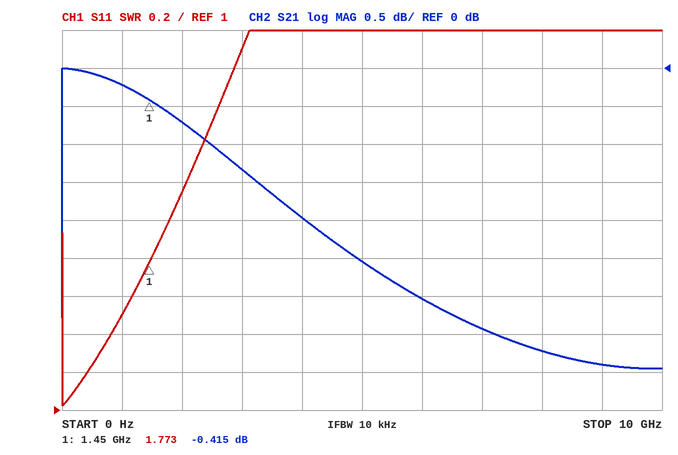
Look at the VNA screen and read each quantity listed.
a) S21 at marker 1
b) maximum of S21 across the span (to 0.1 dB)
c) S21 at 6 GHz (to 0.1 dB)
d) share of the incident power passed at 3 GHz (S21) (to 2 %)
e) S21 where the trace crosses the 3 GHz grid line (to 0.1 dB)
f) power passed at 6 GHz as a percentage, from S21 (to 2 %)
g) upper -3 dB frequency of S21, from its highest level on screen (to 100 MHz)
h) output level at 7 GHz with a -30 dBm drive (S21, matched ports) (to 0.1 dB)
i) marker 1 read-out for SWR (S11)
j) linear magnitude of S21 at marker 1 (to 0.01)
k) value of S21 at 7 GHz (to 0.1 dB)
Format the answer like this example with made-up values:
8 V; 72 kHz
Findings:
-0.415 dB; 0.0 dB; -3.0 dB; 74 %; -1.3 dB; 50 %; 5.9 GHz; -33.4 dBm; 1.773; 0.95; -3.4 dB
